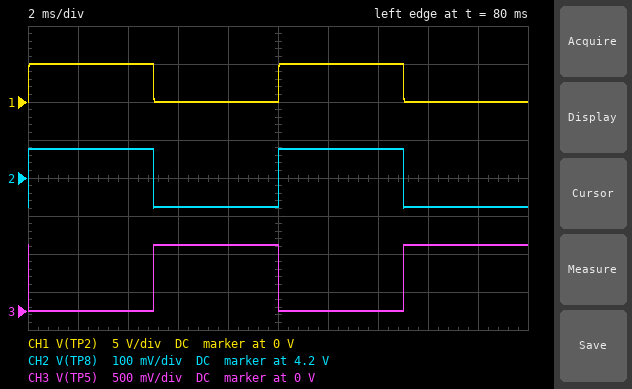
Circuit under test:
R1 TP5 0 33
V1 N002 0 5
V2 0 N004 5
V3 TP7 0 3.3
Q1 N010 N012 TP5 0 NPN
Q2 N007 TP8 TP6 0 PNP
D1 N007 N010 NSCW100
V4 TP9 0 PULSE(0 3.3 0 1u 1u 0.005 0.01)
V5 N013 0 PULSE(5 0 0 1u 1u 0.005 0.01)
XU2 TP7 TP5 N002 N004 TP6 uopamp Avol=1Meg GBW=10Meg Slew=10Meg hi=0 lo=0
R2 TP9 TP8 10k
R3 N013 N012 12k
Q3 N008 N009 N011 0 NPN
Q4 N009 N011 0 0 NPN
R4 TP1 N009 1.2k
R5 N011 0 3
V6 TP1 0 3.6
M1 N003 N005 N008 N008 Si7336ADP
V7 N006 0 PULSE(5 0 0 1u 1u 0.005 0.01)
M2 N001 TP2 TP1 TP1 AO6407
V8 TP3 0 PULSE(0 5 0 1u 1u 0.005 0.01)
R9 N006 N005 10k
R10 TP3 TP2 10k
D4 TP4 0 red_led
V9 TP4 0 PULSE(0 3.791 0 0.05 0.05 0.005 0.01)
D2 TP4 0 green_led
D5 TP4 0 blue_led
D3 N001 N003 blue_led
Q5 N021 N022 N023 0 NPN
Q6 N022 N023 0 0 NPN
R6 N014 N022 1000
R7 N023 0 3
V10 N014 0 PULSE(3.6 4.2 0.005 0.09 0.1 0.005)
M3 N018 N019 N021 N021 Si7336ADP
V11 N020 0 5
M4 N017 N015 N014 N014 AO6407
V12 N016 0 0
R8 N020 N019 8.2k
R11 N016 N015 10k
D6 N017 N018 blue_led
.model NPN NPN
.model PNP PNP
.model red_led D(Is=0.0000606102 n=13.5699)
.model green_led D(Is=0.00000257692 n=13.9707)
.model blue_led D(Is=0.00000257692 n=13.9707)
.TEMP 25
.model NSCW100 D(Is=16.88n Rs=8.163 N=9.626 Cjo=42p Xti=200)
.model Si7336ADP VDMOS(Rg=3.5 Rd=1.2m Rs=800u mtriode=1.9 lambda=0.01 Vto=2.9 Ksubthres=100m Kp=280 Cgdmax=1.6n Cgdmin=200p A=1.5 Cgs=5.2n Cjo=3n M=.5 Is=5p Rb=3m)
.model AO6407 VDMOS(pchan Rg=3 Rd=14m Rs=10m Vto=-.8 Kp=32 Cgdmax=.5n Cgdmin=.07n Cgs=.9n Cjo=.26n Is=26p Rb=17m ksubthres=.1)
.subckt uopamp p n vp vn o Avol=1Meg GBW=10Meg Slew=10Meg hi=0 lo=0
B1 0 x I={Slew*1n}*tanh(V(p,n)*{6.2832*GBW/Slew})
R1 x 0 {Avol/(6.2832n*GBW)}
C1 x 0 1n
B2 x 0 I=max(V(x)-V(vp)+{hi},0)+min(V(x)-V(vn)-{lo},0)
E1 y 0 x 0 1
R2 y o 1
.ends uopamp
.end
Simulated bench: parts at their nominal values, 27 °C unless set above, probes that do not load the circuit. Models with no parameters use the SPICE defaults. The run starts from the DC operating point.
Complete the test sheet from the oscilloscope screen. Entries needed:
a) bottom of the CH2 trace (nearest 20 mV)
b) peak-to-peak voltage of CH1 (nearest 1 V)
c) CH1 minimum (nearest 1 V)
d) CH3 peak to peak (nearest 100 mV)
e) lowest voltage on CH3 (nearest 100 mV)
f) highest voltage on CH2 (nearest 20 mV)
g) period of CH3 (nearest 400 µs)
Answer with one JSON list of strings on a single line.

["4.12 V", "5 V", "0 V", "900 mV", "0 V", "4.28 V", "10.0 ms"]
